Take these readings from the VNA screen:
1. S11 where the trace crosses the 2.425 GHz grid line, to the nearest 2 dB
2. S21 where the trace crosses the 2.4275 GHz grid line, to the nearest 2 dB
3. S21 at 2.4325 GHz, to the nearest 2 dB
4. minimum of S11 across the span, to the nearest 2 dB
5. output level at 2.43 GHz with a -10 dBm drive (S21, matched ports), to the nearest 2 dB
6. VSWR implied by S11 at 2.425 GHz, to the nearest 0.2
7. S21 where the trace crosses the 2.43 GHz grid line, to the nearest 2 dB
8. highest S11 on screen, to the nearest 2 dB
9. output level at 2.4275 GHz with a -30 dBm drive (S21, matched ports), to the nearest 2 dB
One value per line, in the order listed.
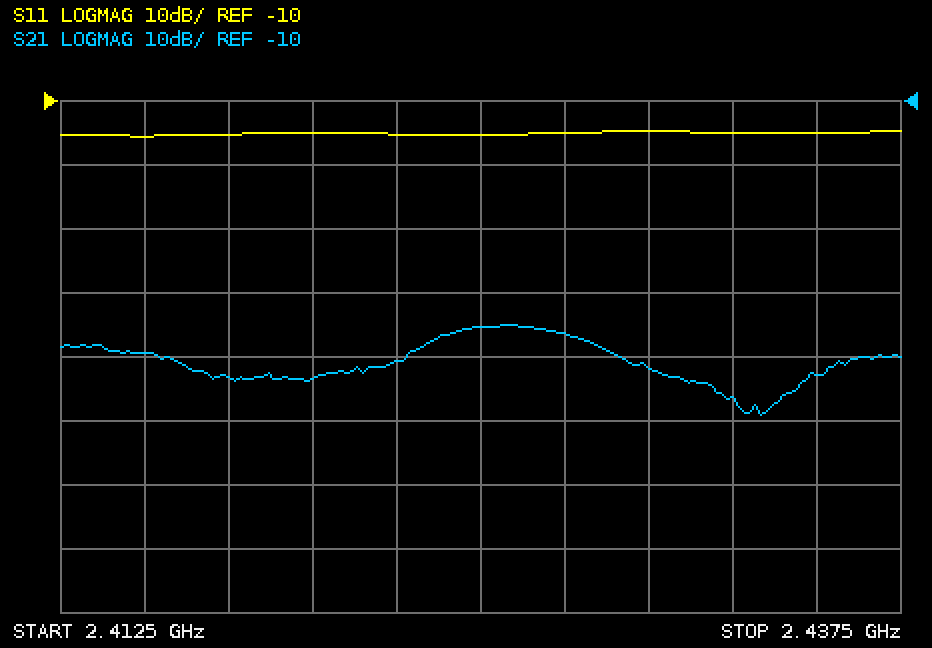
-16 dB
-46 dB
-56 dB
-16 dB
-62 dBm
1.4
-52 dB
-14 dB
-76 dBm
